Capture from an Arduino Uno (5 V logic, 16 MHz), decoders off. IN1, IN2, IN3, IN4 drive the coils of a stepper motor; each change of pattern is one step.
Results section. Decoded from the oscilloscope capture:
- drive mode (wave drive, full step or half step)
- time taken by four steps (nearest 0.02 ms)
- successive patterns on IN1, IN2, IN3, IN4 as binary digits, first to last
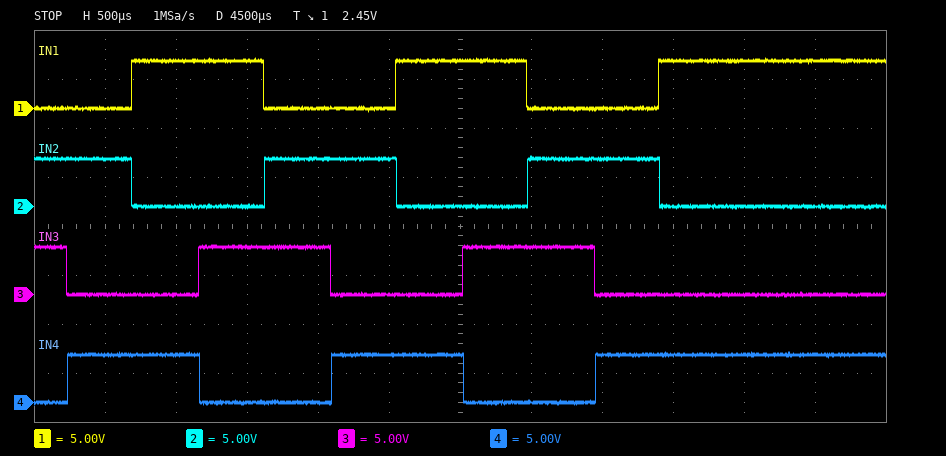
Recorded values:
full step
1.86 ms
0110 0101 1001 1010 0110 0101 1001 1010 0110 0101 1001
